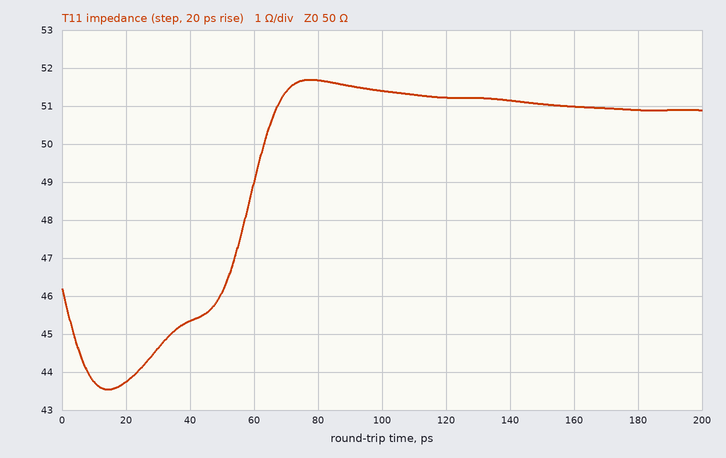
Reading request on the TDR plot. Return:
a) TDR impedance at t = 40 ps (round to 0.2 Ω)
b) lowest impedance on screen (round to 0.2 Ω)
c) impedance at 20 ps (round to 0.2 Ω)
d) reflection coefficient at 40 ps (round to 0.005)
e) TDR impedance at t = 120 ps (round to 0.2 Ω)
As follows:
45.4 Ω
43.6 Ω
43.8 Ω
-0.050
51.2 Ω
